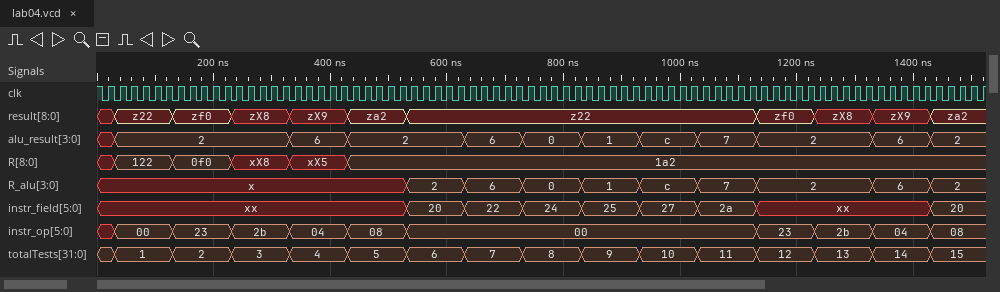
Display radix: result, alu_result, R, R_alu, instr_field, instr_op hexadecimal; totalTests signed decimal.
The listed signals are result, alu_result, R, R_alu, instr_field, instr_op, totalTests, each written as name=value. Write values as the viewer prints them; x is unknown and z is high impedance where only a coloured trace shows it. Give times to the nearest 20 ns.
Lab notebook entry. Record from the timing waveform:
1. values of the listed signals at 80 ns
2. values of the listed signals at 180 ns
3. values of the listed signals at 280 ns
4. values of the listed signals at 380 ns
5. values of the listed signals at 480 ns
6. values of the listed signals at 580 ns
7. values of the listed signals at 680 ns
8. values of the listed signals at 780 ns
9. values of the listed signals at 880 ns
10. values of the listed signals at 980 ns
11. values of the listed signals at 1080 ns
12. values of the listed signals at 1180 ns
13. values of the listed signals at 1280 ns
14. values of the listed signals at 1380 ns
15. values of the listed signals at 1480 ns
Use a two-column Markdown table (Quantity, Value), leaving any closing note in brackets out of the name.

| Quantity | Value |
|---|---|
| values of the listed signals at 80 ns | result=z22, alu_result=2, R=122, R_alu=x, instr_field=xx, instr_op=00, totalTests=1 |
| values of the listed signals at 180 ns | result=zf0, alu_result=2, R=0f0, R_alu=x, instr_field=xx, instr_op=23, totalTests=2 |
| values of the listed signals at 280 ns | result=zX8, alu_result=2, R=xX8, R_alu=x, instr_field=xx, instr_op=2b, totalTests=3 |
| values of the listed signals at 380 ns | result=zX9, alu_result=6, R=xX5, R_alu=x, instr_field=xx, instr_op=04, totalTests=4 |
| values of the listed signals at 480 ns | result=za2, alu_result=2, R=1a2, R_alu=x, instr_field=xx, instr_op=08, totalTests=5 |
| values of the listed signals at 580 ns | result=z22, alu_result=2, R=1a2, R_alu=2, instr_field=20, instr_op=00, totalTests=6 |
| values of the listed signals at 680 ns | result=z22, alu_result=6, R=1a2, R_alu=6, instr_field=22, instr_op=00, totalTests=7 |
| values of the listed signals at 780 ns | result=z22, alu_result=0, R=1a2, R_alu=0, instr_field=24, instr_op=00, totalTests=8 |
| values of the listed signals at 880 ns | result=z22, alu_result=1, R=1a2, R_alu=1, instr_field=25, instr_op=00, totalTests=9 |
| values of the listed signals at 980 ns | result=z22, alu_result=c, R=1a2, R_alu=c, instr_field=27, instr_op=00, totalTests=10 |
| values of the listed signals at 1080 ns | result=z22, alu_result=7, R=1a2, R_alu=7, instr_field=2a, instr_op=00, totalTests=11 |
| values of the listed signals at 1180 ns | result=zf0, alu_result=2, R=1a2, R_alu=2, instr_field=xx, instr_op=23, totalTests=12 |
| values of the listed signals at 1280 ns | result=zX8, alu_result=2, R=1a2, R_alu=2, instr_field=xx, instr_op=2b, totalTests=13 |
| values of the listed signals at 1380 ns | result=zX9, alu_result=6, R=1a2, R_alu=6, instr_field=xx, instr_op=04, totalTests=14 |
| values of the listed signals at 1480 ns | result=za2, alu_result=2, R=1a2, R_alu=2, instr_field=20, instr_op=08, totalTests=15 |
